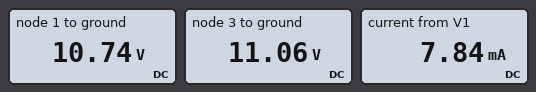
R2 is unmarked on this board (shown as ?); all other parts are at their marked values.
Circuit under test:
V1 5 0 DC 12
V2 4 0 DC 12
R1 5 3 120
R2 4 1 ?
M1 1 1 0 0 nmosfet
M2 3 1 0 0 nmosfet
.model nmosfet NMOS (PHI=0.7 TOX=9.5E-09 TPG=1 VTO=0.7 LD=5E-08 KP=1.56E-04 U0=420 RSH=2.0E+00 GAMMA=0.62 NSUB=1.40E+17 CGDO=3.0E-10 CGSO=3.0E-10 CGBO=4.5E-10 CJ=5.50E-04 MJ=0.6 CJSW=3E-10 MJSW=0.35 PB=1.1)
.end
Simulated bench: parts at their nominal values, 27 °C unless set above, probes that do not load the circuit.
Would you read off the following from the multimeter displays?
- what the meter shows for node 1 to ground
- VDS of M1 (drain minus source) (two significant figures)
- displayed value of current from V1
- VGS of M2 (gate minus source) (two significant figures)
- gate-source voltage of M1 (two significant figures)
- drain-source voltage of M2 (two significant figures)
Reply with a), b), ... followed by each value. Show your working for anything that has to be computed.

a) 10.74 V
b) 10.74 V = 11 V
c) 7.84 mA
d) 10.74 V = 11 V
e) 10.74 V = 11 V
f) 11.06 V = 11 V
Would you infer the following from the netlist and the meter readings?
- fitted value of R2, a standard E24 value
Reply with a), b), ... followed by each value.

a) 160 Ω
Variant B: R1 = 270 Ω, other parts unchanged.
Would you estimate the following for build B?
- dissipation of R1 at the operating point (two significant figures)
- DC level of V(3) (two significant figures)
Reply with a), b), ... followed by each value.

a) 17 mW
b) 9.9 V
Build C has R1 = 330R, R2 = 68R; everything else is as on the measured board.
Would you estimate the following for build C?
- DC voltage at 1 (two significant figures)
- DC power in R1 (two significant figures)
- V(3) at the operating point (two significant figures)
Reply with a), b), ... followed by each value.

a) 11 V
b) 25 mW
c) 9.1 V
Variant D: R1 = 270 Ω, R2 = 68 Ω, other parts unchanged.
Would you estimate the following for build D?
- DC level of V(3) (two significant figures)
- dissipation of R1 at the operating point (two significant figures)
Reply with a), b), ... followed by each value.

a) 9.6 V
b) 21 mW
